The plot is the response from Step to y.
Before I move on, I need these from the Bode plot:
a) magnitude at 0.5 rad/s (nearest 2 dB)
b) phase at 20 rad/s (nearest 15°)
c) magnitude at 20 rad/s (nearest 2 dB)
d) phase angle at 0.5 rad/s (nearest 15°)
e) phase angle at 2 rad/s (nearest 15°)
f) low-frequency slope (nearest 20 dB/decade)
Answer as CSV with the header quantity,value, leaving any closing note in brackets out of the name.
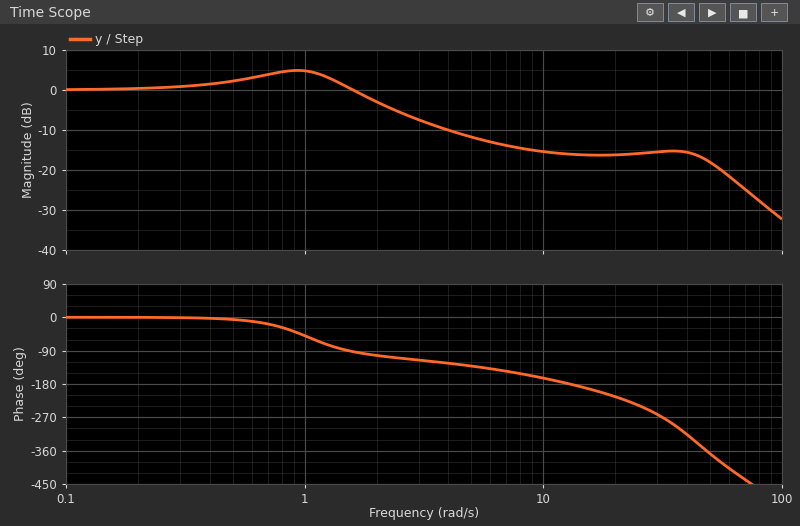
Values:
quantity,value
magnitude at 0.5 rad/s,2 dB
phase at 20 rad/s,-210°
magnitude at 20 rad/s,-16 dB
phase angle at 0.5 rad/s,0°
phase angle at 2 rad/s,-105°
low-frequency slope,0 dB/decade
